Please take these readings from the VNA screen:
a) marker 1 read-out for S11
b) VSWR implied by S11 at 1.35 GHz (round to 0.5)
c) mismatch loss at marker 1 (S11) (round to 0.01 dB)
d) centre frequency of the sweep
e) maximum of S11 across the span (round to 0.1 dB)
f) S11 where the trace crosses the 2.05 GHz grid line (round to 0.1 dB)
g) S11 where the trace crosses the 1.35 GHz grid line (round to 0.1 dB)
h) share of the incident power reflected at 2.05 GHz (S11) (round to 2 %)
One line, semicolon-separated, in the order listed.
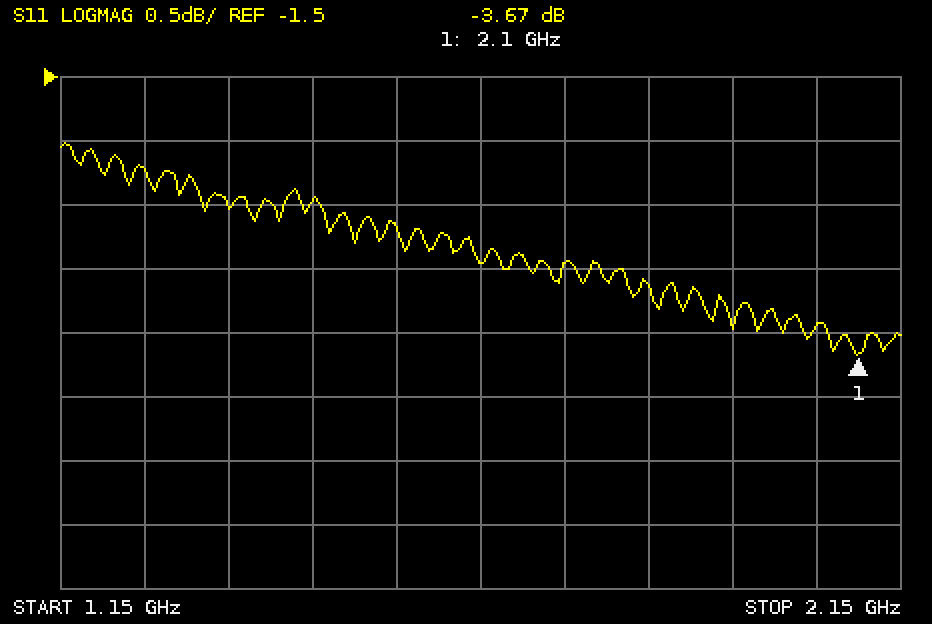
-3.67 dB; 7.0; 2.44 dB; 1.65 GHz; -2.0 dB; -3.4 dB; -2.5 dB; 46 %
